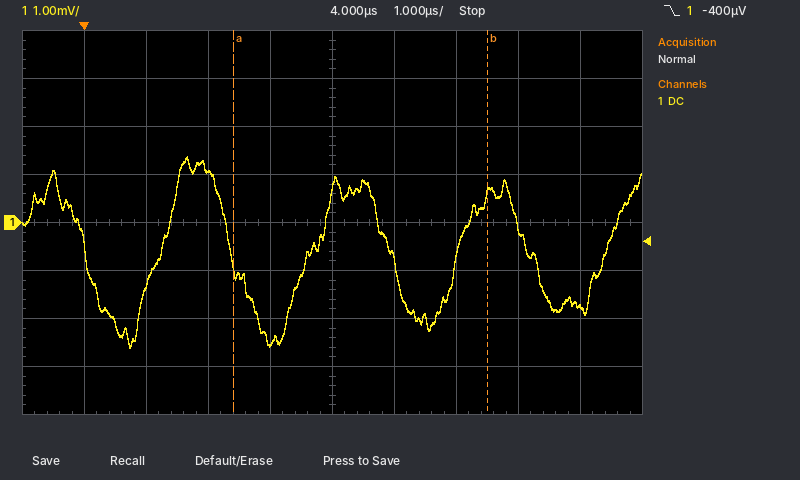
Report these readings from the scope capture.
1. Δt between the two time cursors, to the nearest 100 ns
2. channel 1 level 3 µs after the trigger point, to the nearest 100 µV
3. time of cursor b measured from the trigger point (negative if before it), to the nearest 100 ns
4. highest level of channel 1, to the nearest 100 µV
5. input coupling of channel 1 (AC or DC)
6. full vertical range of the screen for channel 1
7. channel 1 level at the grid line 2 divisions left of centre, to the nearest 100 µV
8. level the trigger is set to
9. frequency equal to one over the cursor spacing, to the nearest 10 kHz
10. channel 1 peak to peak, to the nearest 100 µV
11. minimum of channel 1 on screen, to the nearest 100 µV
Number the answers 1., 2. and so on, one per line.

1. 4.1 µs
2. -2.5 mV
3. +6.5 µs
4. 1.4 mV
5. DC
6. 8 mV
7. 1.1 mV
8. -400 µV
9. 240 kHz
10. 4.0 mV
11. -2.6 mV
